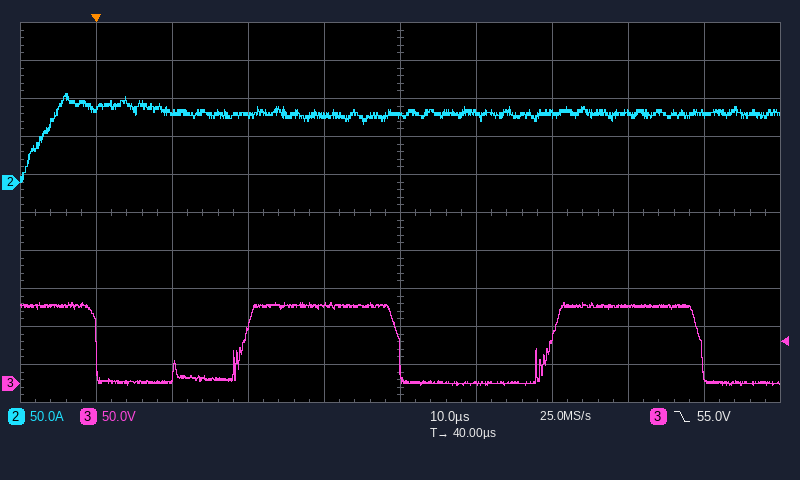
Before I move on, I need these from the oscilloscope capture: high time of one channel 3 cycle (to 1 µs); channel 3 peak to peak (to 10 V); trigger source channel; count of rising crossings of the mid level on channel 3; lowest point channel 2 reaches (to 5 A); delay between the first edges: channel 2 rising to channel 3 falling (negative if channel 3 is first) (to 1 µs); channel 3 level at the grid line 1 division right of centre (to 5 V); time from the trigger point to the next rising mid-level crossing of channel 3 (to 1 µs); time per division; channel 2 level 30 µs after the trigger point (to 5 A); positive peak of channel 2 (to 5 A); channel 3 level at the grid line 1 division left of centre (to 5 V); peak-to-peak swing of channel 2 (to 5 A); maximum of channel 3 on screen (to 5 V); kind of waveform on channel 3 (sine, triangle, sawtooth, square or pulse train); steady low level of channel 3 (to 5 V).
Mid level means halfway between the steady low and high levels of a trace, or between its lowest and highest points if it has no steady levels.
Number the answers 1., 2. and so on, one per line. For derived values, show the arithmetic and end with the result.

1. 20 µs
2. 110 V
3. channel 3
4. 2
5. 0 A
6. +7 µs
7. 0 V
8. 19 µs
9. 10 µs
10. 90 A
11. 115 A
12. 105 V
13. 115 A − (0 A) = 115 A
14. 105 V
15. square
16. 0 V
